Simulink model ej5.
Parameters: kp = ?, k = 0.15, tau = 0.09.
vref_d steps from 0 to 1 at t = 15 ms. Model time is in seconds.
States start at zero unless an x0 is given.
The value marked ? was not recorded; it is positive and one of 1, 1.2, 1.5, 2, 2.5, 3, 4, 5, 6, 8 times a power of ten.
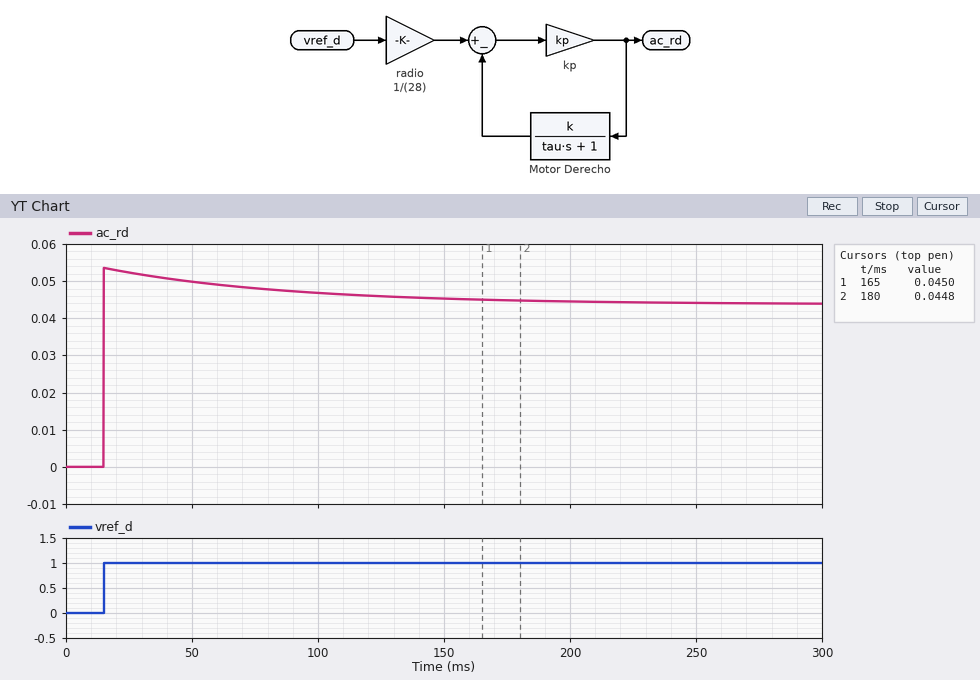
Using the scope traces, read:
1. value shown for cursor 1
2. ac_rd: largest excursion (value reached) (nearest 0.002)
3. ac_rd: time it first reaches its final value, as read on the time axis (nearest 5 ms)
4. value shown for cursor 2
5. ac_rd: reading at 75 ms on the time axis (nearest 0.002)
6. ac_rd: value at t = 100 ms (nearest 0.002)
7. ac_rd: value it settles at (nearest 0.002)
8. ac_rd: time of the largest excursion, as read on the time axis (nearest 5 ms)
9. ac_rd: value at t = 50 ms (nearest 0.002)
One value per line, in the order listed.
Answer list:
0.0450
0.054
15 ms
0.0448
0.048
0.046
0.044
15 ms
0.050
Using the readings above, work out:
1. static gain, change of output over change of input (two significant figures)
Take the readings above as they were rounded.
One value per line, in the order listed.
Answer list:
0.044
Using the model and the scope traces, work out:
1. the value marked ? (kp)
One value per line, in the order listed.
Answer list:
1.5
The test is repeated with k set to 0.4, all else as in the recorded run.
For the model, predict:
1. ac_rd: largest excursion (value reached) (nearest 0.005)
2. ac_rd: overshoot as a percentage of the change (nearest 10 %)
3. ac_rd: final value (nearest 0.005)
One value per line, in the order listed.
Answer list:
0.055
60 %
0.035
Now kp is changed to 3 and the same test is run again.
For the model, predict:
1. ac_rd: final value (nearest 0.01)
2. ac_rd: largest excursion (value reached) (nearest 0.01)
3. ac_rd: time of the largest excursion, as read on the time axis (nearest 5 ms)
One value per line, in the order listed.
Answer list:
0.07
0.11
15 ms
